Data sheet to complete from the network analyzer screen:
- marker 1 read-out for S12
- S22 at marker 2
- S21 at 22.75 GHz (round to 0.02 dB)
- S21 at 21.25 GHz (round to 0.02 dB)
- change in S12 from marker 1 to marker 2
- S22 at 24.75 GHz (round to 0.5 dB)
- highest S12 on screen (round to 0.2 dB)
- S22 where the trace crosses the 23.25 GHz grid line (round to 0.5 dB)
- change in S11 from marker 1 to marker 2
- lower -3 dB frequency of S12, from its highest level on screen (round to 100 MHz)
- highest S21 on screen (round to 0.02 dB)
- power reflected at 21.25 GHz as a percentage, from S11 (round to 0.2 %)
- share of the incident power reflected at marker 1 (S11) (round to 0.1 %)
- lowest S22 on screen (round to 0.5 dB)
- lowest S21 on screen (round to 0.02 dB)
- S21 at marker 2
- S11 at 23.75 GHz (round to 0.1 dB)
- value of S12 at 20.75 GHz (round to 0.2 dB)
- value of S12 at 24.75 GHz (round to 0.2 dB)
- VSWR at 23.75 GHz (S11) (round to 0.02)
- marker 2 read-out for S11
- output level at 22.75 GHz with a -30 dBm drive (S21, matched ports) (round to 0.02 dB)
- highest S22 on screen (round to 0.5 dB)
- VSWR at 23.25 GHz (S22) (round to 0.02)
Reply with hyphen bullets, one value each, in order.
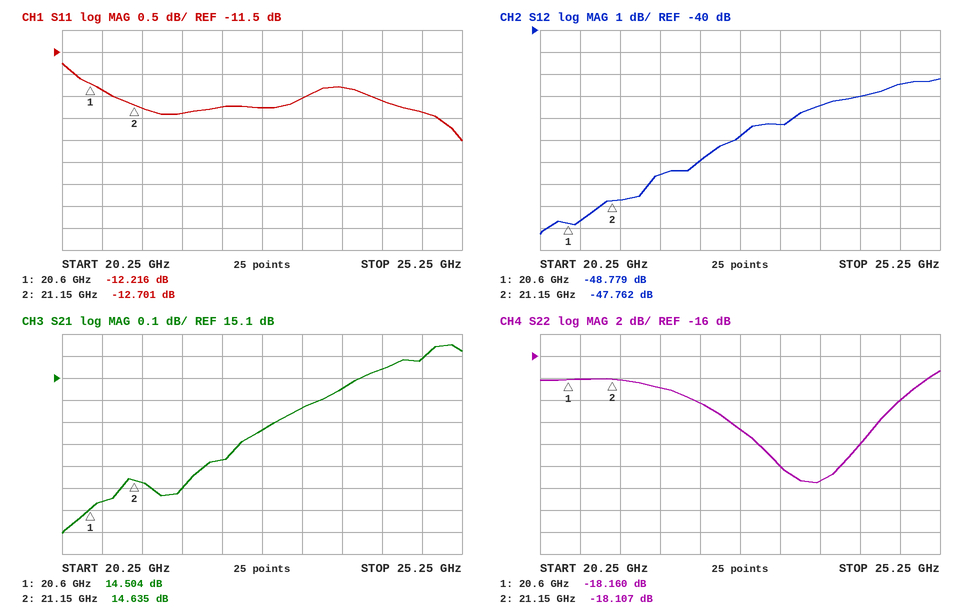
- -48.779 dB
- -18.107 dB
- 14.86 dB
- 14.62 dB
- 1.017 dB
- -20.0 dB
- -42.2 dB
- -26.0 dB
- -0.485 dB
- 22.5 GHz
- 15.26 dB
- 5.2 %
- 6.0 %
- -27.5 dB
- 14.40 dB
- 14.635 dB
- -12.3 dB
- -48.6 dB
- -42.4 dB
- 1.64
- -12.701 dB
- -15.14 dBm
- -17.5 dB
- 1.10
